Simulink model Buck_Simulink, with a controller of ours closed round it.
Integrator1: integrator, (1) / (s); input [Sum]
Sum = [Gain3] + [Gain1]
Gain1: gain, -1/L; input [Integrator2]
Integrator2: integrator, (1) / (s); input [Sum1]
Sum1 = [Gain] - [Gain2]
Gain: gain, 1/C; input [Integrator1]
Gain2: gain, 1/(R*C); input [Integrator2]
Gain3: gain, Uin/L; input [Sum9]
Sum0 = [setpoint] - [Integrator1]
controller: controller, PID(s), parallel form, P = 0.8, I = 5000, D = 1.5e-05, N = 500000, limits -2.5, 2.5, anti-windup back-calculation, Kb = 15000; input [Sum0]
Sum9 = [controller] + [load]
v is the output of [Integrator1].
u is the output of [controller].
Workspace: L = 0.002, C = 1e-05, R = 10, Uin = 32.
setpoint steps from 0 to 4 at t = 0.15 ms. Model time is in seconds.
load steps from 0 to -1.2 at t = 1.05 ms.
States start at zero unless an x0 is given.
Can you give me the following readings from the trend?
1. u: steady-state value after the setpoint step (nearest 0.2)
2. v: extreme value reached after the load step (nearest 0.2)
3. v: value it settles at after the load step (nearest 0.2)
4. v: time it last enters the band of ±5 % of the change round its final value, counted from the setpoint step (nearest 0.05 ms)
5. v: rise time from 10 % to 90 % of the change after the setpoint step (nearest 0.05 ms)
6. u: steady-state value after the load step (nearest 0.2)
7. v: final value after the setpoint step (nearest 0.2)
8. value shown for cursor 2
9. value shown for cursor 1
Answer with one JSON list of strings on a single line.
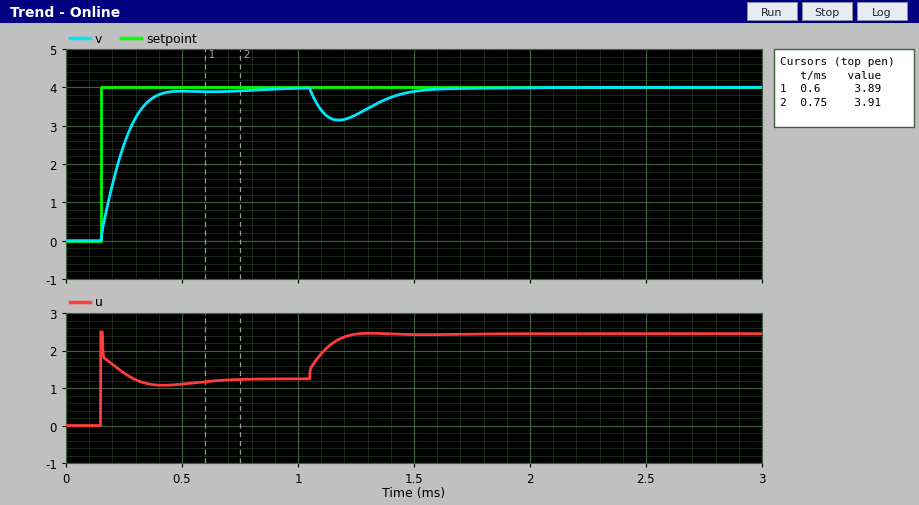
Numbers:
["1.2", "3.2", "4.0", "0.25 ms", "0.20 ms", "2.4", "4.0", "3.91", "3.89"]
